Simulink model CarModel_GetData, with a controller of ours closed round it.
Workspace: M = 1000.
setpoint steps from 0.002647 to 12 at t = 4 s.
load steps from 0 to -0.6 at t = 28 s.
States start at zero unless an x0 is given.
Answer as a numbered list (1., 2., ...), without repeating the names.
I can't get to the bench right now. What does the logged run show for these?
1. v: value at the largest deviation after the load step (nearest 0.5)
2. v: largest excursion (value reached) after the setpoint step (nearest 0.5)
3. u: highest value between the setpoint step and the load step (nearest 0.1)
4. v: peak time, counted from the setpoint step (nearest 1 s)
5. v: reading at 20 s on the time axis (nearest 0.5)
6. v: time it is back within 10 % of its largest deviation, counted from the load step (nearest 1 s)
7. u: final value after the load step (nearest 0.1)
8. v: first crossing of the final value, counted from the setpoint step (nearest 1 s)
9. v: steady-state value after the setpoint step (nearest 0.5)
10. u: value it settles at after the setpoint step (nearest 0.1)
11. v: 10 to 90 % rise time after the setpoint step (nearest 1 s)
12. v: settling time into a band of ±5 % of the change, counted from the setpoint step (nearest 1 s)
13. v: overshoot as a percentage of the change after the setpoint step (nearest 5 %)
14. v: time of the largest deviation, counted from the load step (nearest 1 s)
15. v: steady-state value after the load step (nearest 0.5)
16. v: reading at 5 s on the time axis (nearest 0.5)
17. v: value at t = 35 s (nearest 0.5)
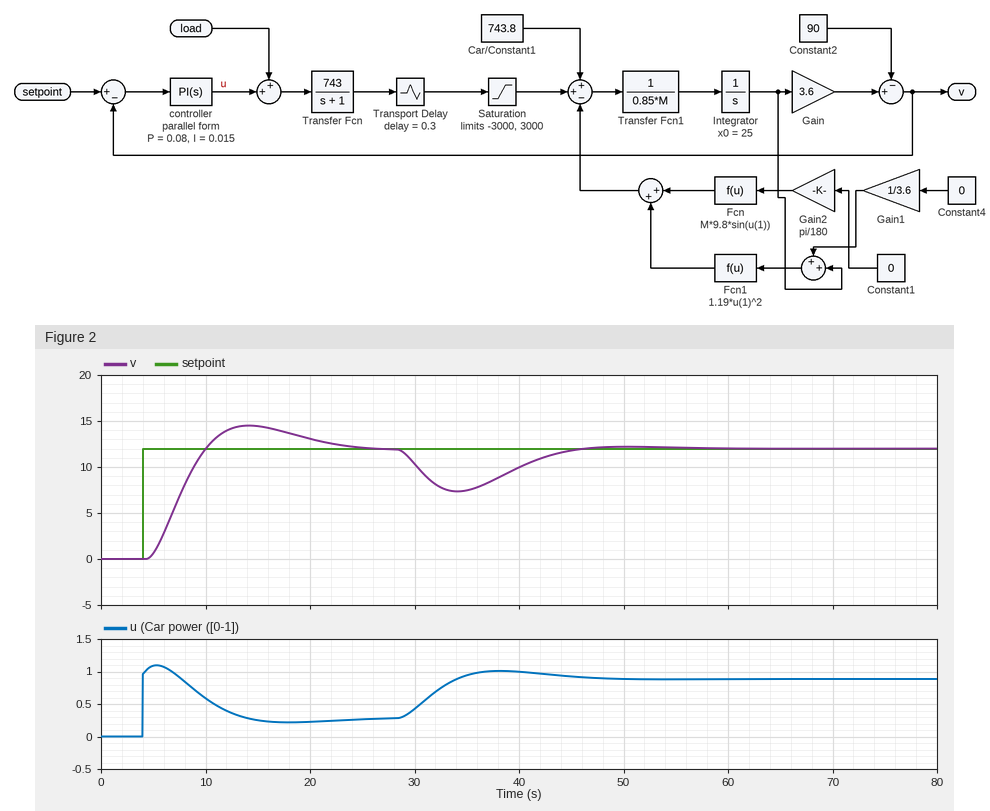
1. 7.5
2. 14.5
3. 1.1
4. 10 s
5. 13.0
6. 16 s
7. 0.9
8. 6 s
9. 12.0
10. 0.3
11. 4 s
12. 18 s
13. 20 %
14. 6 s
15. 12.0
16. 0.5
17. 7.5
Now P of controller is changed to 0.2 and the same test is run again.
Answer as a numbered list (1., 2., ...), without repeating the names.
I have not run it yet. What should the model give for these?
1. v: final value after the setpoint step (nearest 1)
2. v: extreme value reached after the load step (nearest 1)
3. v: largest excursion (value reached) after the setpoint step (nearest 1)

1. 12
2. 9
3. 14
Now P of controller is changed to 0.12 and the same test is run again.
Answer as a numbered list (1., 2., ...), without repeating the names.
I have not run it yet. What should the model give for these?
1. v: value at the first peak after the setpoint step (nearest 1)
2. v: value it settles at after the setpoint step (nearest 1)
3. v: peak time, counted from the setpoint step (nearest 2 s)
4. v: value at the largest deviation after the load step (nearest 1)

1. 14
2. 12
3. 8 s
4. 8
